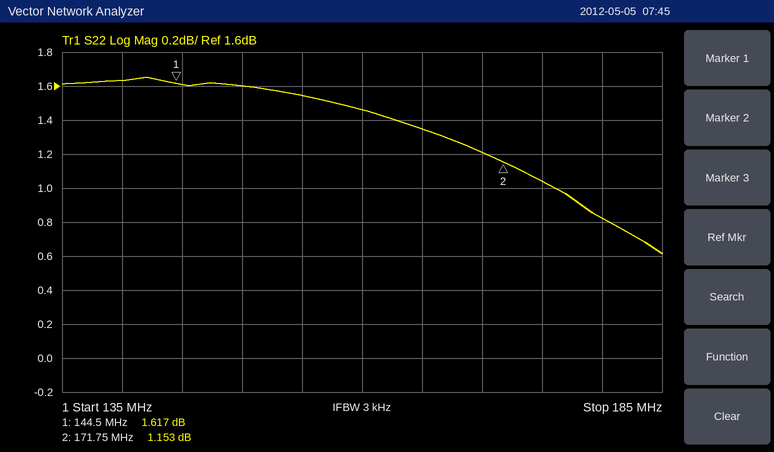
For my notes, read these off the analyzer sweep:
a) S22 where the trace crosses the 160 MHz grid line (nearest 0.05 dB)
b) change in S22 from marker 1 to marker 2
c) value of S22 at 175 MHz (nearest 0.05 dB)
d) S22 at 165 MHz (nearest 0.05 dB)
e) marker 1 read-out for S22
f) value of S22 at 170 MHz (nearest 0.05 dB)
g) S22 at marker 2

1.45 dB
-0.464 dB
1.05 dB
1.35 dB
1.617 dB
1.20 dB
1.153 dB
